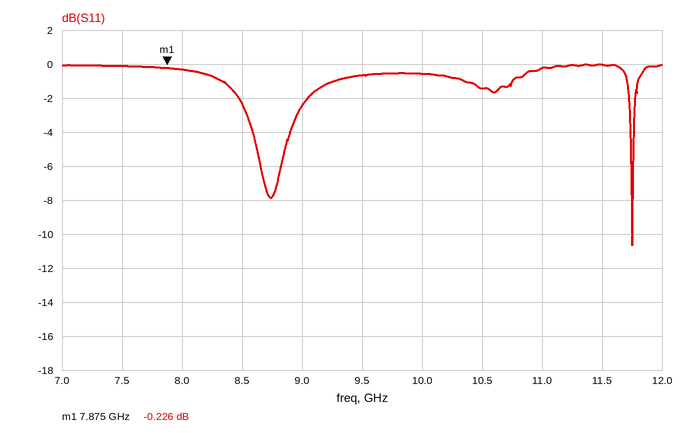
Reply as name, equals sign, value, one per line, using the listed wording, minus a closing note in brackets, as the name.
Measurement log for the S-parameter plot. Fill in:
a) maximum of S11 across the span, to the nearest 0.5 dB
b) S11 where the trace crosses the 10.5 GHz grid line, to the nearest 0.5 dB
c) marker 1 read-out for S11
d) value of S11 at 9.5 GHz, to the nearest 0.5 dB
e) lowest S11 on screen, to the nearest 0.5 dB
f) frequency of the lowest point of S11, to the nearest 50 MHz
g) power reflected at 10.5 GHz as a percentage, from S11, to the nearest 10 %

maximum of S11 across the span, to the nearest 0.5 dB = 0.0 dB
S11 where the trace crosses the 10.5 GHz grid line, to the nearest 0.5 dB = -1.5 dB
marker 1 read-out for S11 = -0.226 dB
value of S11 at 9.5 GHz, to the nearest 0.5 dB = -0.5 dB
lowest S11 on screen, to the nearest 0.5 dB = -10.5 dB
frequency of the lowest point of S11, to the nearest 50 MHz = 11.75 GHz
power reflected at 10.5 GHz as a percentage, from S11, to the nearest 10 % = 70 %
